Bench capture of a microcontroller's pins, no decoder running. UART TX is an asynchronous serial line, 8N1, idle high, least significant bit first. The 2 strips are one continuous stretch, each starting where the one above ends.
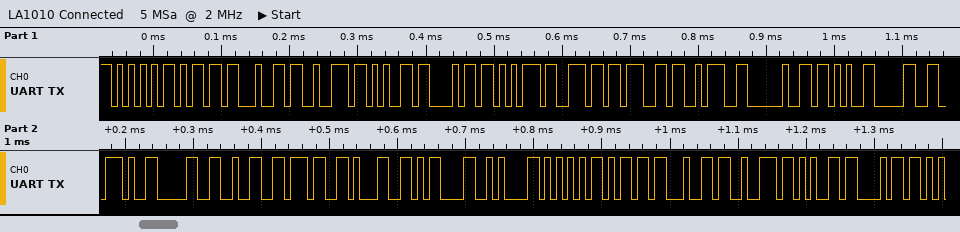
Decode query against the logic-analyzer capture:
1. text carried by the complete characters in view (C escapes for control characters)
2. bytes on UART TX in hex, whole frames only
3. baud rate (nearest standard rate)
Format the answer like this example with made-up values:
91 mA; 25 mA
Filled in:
"Umdrehung: +0.0271\r\nUmdreh"; 55 6D 64 72 65 68 75 6E 67 3A 20 2B 30 2E 30 32 37 31 0D 0A 55 6D 64 72 65 68; 115200 baud
